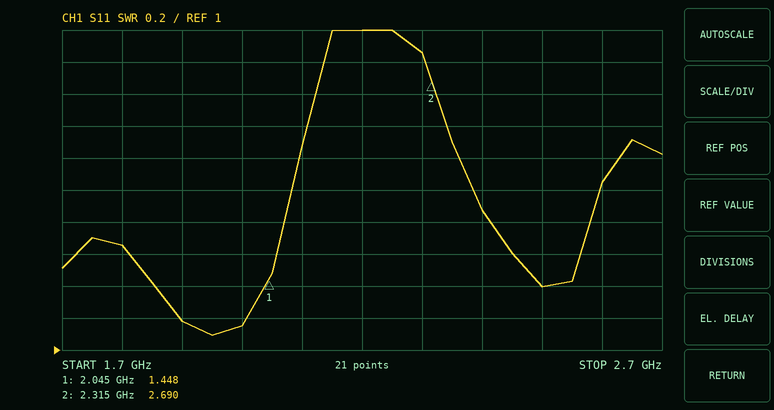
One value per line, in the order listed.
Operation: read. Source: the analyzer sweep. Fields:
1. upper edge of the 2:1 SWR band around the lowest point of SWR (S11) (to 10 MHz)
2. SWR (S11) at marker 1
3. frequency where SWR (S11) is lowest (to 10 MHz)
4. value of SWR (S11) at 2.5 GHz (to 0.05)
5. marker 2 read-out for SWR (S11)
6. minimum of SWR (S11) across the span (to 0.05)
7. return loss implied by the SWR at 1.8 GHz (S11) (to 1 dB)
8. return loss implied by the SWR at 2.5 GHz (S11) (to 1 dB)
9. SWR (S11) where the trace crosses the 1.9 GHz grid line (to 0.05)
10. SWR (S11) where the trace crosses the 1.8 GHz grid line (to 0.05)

2.08 GHz
1.448
1.95 GHz
1.40
2.690
1.10
12 dB
16 dB
1.20
1.65
